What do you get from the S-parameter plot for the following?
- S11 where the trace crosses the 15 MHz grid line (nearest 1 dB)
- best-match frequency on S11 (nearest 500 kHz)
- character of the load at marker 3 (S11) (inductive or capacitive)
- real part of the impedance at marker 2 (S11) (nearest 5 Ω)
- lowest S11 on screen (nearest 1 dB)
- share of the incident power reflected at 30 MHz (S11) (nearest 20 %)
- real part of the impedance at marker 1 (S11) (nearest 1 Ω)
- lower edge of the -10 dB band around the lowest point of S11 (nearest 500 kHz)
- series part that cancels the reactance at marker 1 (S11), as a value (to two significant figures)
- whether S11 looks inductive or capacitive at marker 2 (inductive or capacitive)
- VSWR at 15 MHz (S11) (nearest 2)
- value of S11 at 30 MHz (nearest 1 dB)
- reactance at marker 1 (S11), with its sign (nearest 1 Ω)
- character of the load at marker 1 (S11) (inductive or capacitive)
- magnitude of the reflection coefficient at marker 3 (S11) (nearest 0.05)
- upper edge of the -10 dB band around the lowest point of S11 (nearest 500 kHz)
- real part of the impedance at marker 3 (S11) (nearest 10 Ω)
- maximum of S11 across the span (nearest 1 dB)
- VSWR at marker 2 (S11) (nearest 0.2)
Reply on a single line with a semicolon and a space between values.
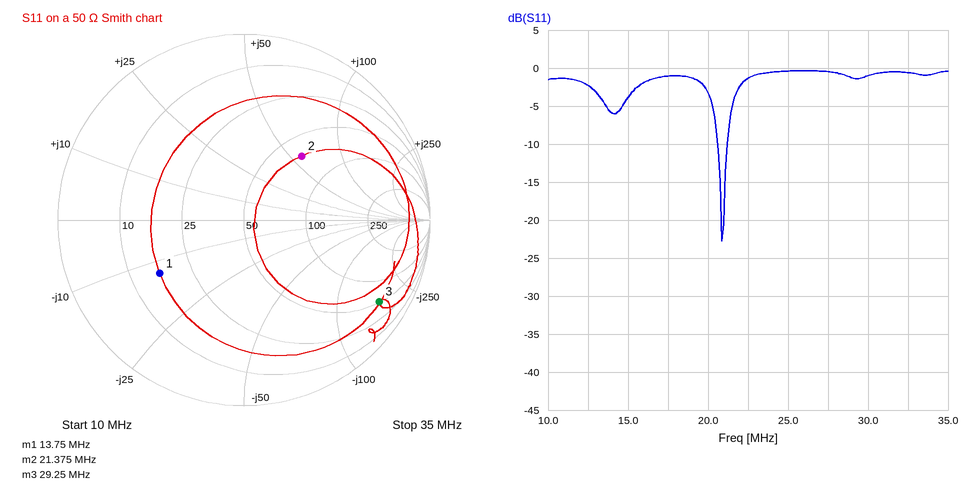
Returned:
-4 dB; 21.0 MHz; capacitive; 65 Ω; -23 dB; 80 %; 16 Ω; 20.5 MHz; 150 nH; inductive; 4; -1 dB; -13 Ω; capacitive; 0.85; 21.0 MHz; 50 Ω; 0 dB; 2.8
